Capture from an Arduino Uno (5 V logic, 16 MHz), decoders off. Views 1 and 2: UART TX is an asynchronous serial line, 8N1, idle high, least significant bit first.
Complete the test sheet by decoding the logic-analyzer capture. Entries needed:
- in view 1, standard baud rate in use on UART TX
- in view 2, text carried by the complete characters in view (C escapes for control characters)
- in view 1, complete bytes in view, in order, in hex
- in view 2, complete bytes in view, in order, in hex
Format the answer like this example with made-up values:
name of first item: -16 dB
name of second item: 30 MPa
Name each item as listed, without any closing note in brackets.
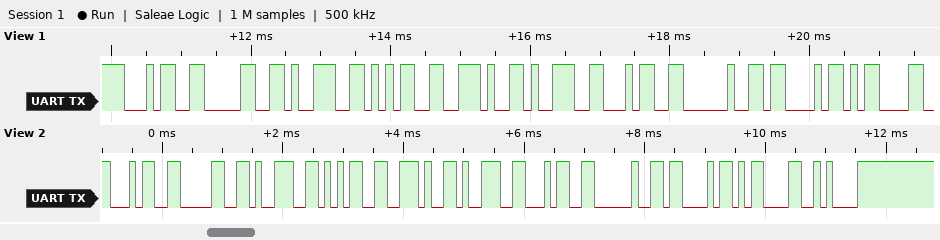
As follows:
in view 1, standard baud rate in use on UART TX: 9600 baud
in view 2, text carried by the complete characters in view: "4095.94 C\r\n"
in view 1, complete bytes in view, in order, in hex: 0x34 0x30 0x39 0x35 0x2E 0x39 0x34 0x20 0x43 0x0D
in view 2, complete bytes in view, in order, in hex: 34 30 39 35 2E 39 34 20 43 0D 0A
